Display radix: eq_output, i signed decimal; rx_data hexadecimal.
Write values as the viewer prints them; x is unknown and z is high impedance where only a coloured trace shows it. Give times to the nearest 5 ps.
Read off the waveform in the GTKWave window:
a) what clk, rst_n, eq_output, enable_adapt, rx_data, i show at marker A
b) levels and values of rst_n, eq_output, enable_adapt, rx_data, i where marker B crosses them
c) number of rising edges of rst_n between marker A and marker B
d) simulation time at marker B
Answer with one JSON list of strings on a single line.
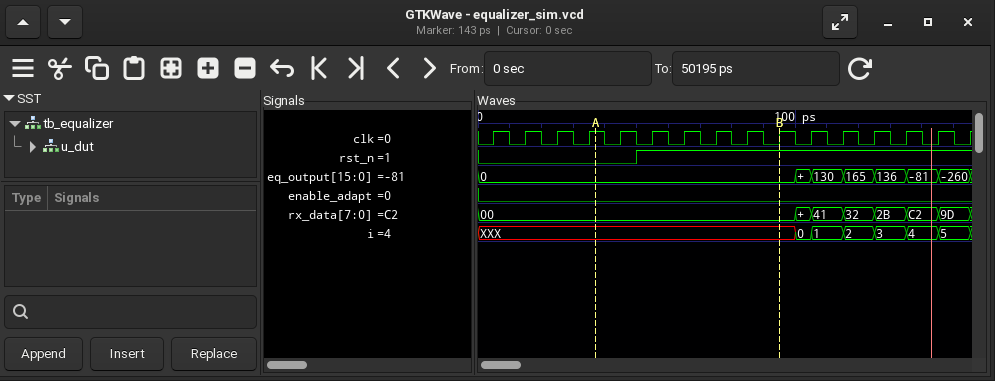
["clk=1, rst_n=0, eq_output=0, enable_adapt=0, rx_data=00, i=XXX", "rst_n=1, eq_output=0, enable_adapt=0, rx_data=00, i=XXX", "1", "95 ps"]
